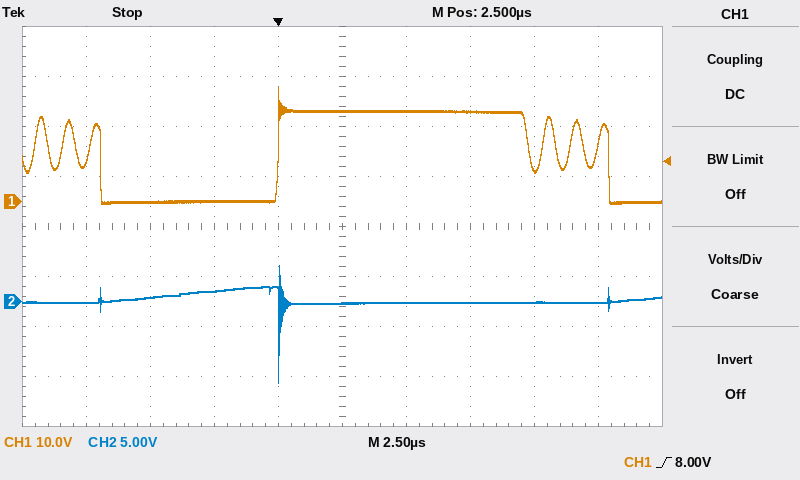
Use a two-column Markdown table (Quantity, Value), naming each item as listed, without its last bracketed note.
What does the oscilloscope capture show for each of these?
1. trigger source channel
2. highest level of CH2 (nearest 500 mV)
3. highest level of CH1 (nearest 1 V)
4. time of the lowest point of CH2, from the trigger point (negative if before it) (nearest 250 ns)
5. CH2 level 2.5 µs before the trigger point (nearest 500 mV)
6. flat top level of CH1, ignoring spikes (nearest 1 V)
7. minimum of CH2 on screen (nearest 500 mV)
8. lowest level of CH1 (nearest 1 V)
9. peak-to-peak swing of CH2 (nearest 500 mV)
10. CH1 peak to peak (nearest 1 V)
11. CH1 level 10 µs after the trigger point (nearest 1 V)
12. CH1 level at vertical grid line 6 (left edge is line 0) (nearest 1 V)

| Quantity | Value |
|---|---|
| trigger source channel | CH1 |
| highest level of CH2 | 3.5 V |
| highest level of CH1 | 23 V |
| time of the lowest point of CH2, from the trigger point (negative if before it) | 0.00 µs |
| CH2 level 2.5 µs before the trigger point | 1.0 V |
| flat top level of CH1, ignoring spikes | 18 V |
| minimum of CH2 on screen | -8.0 V |
| lowest level of CH1 | 0 V |
| peak-to-peak swing of CH2 | 11.5 V |
| CH1 peak to peak | 23 V |
| CH1 level 10 µs after the trigger point | 7 V |
| CH1 level at vertical grid line 6 (left edge is line 0) | 18 V |
